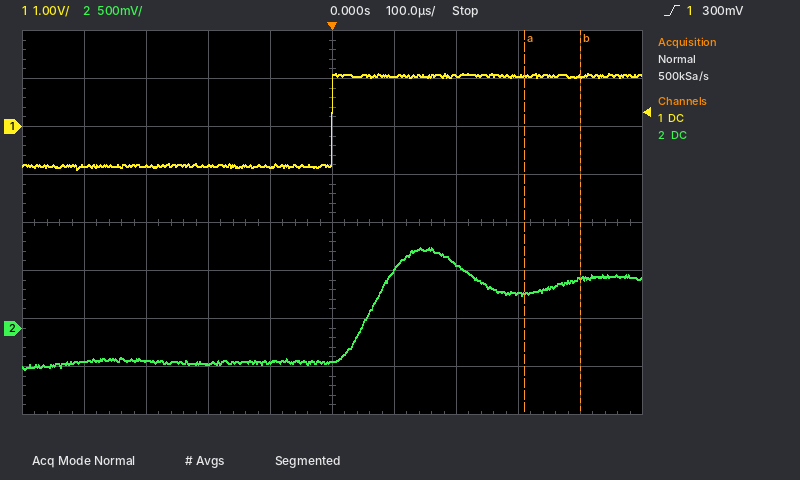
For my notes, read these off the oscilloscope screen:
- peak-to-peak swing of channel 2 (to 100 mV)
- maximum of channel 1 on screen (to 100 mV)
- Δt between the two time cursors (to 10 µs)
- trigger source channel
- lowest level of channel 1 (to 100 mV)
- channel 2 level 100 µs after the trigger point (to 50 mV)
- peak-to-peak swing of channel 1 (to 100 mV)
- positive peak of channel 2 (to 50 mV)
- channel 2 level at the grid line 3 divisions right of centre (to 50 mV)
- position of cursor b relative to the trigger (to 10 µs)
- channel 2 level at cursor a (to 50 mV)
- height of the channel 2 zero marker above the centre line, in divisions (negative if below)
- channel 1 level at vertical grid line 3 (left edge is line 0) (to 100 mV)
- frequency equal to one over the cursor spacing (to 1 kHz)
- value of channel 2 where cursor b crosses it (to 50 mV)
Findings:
1.30 V
1.1 V
90 µs
channel 1
-900 mV
600 mV
2.0 V
850 mV
350 mV
+400 µs
350 mV
-2.2 div
-800 mV
11 kHz
500 mV
